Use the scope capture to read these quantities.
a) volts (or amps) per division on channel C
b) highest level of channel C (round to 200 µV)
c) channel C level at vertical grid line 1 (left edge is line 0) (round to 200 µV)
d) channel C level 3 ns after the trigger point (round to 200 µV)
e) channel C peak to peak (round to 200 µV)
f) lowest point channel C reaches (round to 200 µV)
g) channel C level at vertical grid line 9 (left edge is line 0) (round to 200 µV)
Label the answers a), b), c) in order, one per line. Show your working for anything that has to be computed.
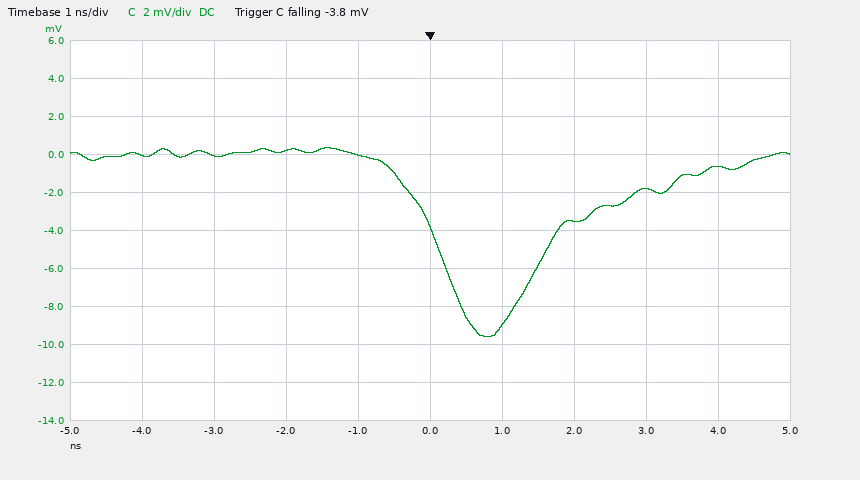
a) 2 mV
b) 400 µV
c) 0.0 mV
d) -1.8 mV
e) 400 µV − (-9.6 mV) = 10.0 mV
f) -9.6 mV
g) -600 µV
